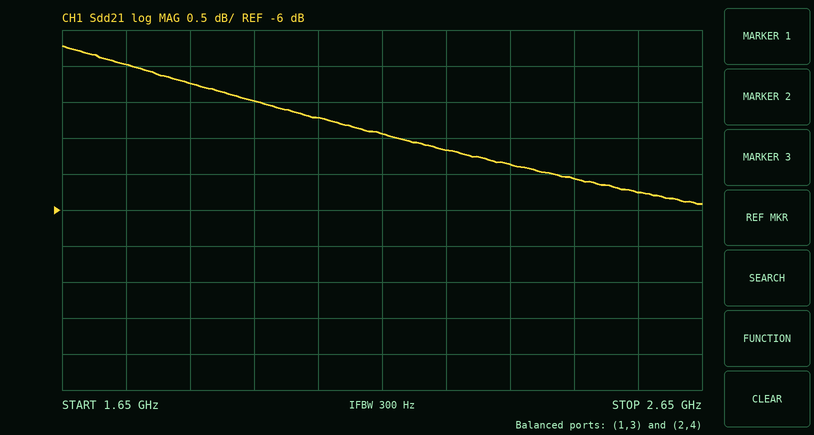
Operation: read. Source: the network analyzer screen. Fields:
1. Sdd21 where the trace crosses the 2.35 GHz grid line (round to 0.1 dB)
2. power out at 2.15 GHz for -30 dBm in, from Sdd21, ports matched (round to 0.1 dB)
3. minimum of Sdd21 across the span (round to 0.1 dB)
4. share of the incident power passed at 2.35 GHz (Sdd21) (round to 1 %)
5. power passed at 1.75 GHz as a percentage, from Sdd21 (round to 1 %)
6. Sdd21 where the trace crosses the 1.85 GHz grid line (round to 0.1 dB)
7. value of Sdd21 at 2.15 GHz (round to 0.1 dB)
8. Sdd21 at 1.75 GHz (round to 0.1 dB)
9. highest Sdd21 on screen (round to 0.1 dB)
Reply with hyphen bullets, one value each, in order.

- -5.4 dB
- -34.9 dBm
- -5.9 dB
- 29 %
- 40 %
- -4.2 dB
- -4.9 dB
- -4.0 dB
- -3.7 dB
